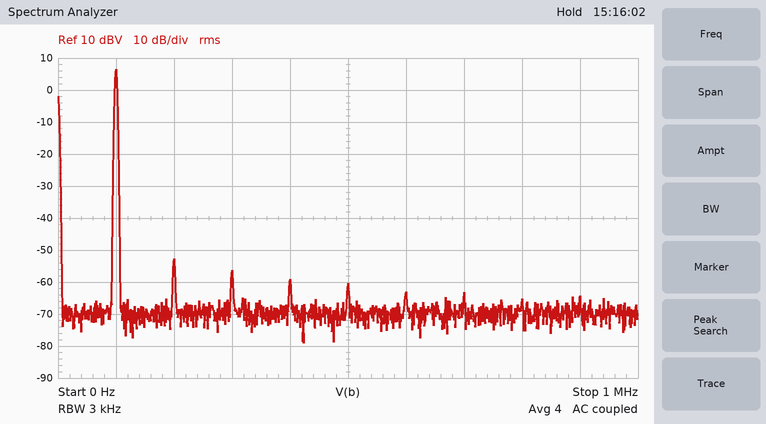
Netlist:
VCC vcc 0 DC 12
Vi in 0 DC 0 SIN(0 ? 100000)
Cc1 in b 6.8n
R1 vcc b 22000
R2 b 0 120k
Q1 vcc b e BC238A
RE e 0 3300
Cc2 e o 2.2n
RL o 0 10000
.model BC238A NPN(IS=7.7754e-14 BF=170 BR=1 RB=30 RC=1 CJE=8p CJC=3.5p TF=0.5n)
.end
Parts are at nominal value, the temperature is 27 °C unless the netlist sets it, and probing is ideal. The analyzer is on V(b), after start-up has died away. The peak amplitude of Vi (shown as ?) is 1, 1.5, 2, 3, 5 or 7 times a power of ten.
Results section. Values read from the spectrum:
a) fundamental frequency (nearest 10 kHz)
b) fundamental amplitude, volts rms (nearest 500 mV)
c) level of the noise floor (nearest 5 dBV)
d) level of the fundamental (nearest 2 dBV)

100 kHz
2.0 V
-70 dBV
6 dBV
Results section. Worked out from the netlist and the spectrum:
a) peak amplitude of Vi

3 V
